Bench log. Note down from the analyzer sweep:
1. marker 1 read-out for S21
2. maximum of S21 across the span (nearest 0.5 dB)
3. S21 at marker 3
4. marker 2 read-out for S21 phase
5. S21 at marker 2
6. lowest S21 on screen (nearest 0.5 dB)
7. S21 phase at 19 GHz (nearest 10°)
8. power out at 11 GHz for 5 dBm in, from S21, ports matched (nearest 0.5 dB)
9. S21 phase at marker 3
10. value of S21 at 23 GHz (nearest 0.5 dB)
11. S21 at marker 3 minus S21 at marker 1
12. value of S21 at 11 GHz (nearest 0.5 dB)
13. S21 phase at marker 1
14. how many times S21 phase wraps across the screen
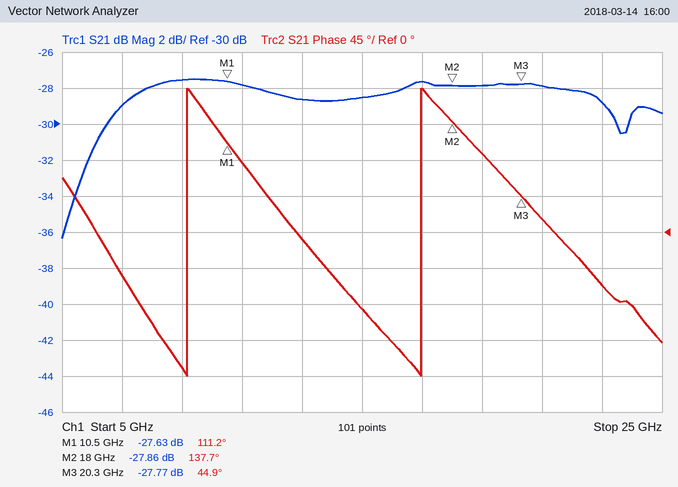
-27.63 dB
-27.5 dB
-27.77 dB
137.7°
-27.86 dB
-36.5 dB
100°
-23.0 dBm
44.9°
-29.0 dB
-0.14 dB
-28.0 dB
111.2°
2
